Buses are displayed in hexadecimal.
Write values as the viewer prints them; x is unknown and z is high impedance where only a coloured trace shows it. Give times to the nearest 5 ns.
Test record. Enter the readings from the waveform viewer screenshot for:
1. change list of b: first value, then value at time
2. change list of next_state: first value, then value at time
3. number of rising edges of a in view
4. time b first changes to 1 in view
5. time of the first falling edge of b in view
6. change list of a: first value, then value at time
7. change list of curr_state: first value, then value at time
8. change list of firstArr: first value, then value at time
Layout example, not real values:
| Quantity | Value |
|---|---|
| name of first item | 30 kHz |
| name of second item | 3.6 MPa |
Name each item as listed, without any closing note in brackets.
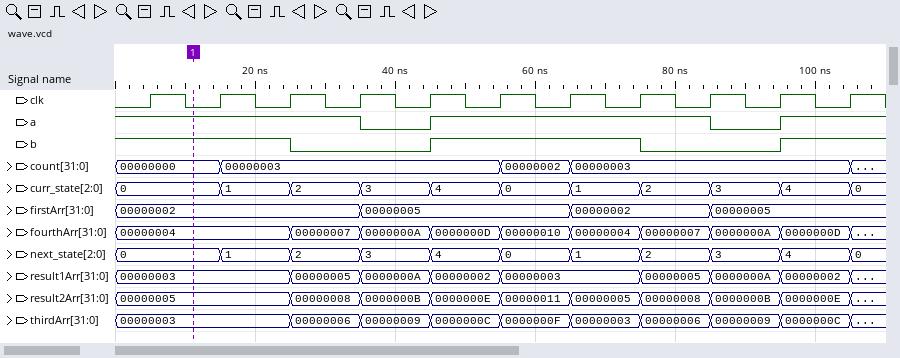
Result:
| Quantity | Value |
|---|---|
| change list of b: first value, then value at time | 1, 0 at 25 ns, 1 at 45 ns, 0 at 75 ns, 1 at 95 ns |
| change list of next_state: first value, then value at time | 0, 1 at 15 ns, 2 at 25 ns, 3 at 35 ns, 4 at 45 ns, 0 at 55 ns, 1 at 65 ns, 2 at 75 ns, 3 at 85 ns, 4 at 95 ns, 0 at 105 ns |
| number of rising edges of a in view | 2 |
| time b first changes to 1 in view | 45 ns |
| time of the first falling edge of b in view | 25 ns |
| change list of a: first value, then value at time | 1, 0 at 35 ns, 1 at 45 ns, 0 at 85 ns, 1 at 95 ns |
| change list of curr_state: first value, then value at time | 0, 1 at 15 ns, 2 at 25 ns, 3 at 35 ns, 4 at 45 ns, 0 at 55 ns, 1 at 65 ns, 2 at 75 ns, 3 at 85 ns, 4 at 95 ns, 0 at 105 ns |
| change list of firstArr: first value, then value at time | 00000002, 00000005 at 35 ns, 00000002 at 65 ns, 00000005 at 85 ns |
